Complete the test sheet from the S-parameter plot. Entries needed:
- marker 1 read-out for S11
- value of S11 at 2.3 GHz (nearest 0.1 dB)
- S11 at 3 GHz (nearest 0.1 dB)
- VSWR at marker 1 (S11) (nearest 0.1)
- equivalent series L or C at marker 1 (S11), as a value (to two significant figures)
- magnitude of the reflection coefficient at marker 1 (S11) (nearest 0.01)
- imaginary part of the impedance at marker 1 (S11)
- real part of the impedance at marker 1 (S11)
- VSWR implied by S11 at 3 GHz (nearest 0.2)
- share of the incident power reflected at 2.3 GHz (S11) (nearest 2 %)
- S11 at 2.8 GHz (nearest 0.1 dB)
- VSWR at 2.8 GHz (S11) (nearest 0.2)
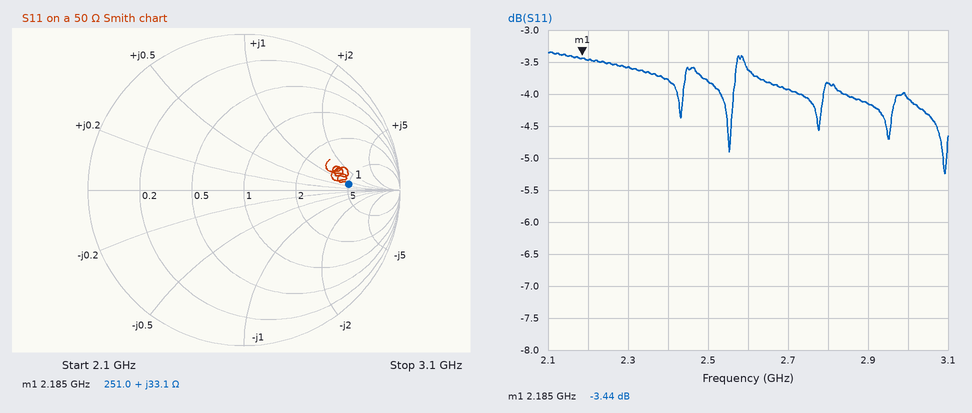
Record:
-3.44 dB
-3.6 dB
-4.1 dB
5.1
2.4 nH
0.67
+33.1 Ω
251.0 Ω
4.4
44 %
-3.8 dB
4.6
